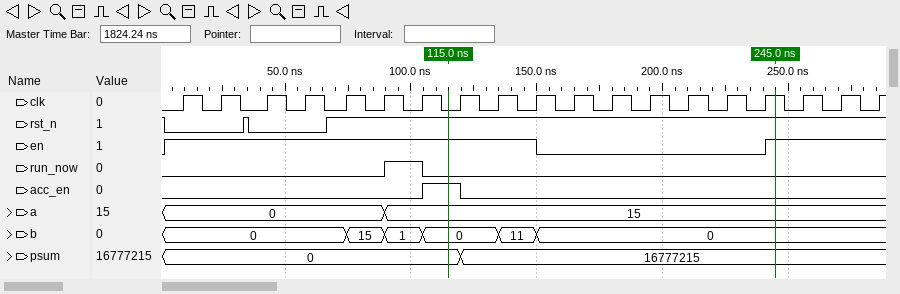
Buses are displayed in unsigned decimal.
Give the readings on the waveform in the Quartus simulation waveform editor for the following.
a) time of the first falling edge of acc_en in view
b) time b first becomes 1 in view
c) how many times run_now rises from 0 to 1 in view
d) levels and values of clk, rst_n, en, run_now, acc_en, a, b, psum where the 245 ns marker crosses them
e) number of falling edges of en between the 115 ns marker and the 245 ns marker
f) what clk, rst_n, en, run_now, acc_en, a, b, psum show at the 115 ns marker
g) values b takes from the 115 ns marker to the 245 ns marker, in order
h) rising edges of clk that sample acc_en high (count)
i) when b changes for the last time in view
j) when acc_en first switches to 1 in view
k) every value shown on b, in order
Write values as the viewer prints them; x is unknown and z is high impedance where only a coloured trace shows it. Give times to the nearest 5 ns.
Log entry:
120 ns
90 ns
1
clk=1, rst_n=1, en=1, run_now=0, acc_en=0, a=15, b=0, psum=16777215
1
clk=0, rst_n=1, en=1, run_now=0, acc_en=1, a=15, b=0, psum=0
0, 11, 0
1
150 ns
105 ns
0, 15, 1, 0, 11, 0
